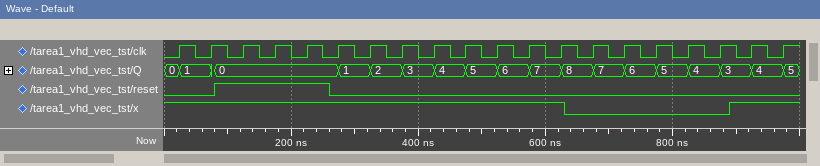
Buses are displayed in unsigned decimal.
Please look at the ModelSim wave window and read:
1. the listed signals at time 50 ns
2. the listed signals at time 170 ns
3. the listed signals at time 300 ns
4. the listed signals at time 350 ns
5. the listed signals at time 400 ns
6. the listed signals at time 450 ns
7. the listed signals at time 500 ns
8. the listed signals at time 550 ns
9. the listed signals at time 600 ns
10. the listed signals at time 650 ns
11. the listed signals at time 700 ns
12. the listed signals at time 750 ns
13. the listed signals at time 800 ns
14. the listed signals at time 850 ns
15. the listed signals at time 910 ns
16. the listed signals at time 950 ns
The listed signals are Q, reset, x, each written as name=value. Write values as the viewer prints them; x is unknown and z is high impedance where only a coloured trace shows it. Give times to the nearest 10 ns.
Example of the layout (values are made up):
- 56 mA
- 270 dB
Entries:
- Q=1, reset=0, x=1
- Q=0, reset=1, x=1
- Q=1, reset=0, x=1
- Q=2, reset=0, x=1
- Q=3, reset=0, x=1
- Q=4, reset=0, x=1
- Q=5, reset=0, x=1
- Q=6, reset=0, x=1
- Q=7, reset=0, x=1
- Q=8, reset=0, x=0
- Q=7, reset=0, x=0
- Q=6, reset=0, x=0
- Q=5, reset=0, x=0
- Q=4, reset=0, x=0
- Q=3, reset=0, x=1
- Q=4, reset=0, x=1
